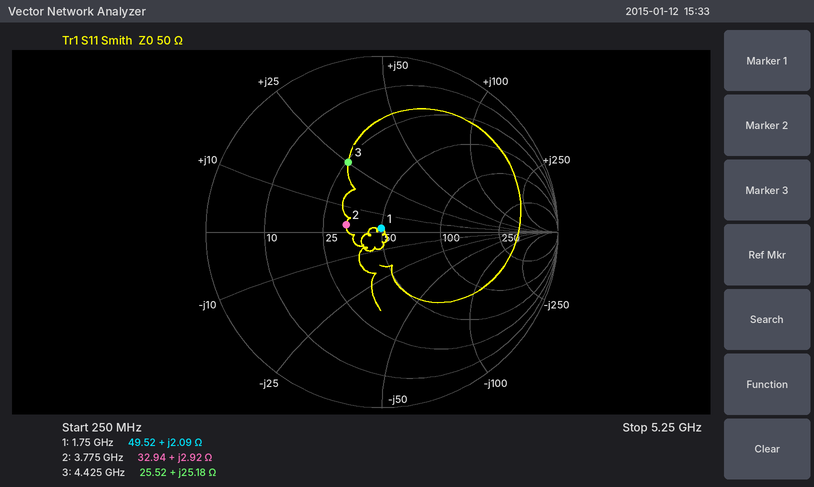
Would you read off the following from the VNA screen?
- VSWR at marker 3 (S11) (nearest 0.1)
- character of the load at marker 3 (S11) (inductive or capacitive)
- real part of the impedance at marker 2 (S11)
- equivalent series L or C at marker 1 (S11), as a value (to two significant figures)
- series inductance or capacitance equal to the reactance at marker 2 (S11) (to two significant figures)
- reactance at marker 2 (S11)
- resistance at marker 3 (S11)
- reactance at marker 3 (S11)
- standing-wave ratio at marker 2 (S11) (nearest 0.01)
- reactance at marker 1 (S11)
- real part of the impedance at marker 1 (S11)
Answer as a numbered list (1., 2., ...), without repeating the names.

1. 2.6
2. inductive
3. 32.94 Ω
4. 190 pH
5. 120 pH
6. +2.92 Ω
7. 25.52 Ω
8. +25.18 Ω
9. 1.53
10. +2.09 Ω
11. 49.52 Ω
